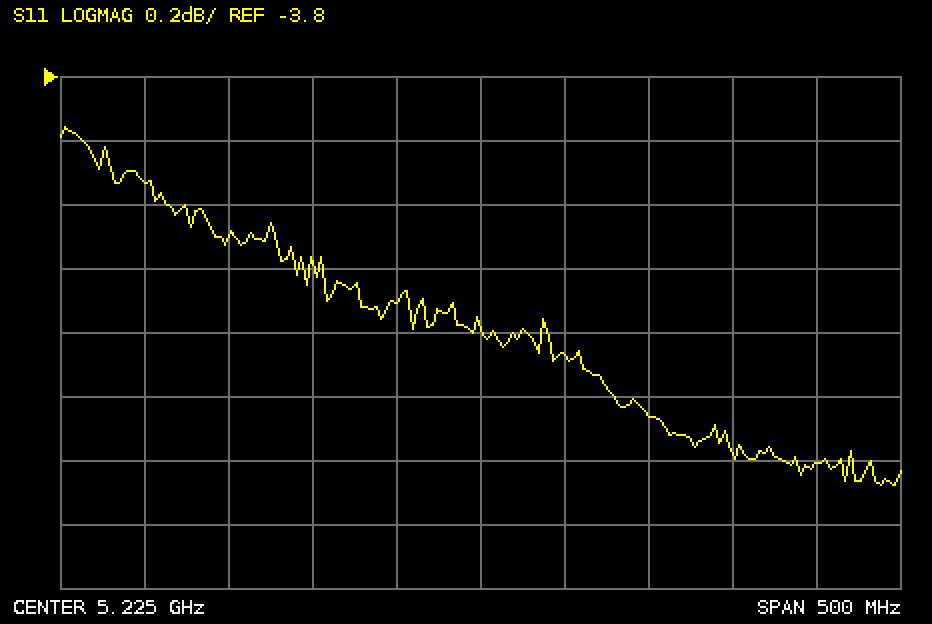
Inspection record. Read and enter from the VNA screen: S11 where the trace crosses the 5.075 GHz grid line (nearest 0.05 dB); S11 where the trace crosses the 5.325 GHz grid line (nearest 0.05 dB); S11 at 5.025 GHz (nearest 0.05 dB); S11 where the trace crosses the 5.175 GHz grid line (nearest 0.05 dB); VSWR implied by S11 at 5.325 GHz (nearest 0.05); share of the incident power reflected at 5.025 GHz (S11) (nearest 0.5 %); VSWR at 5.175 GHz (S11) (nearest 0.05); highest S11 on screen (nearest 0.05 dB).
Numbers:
-4.30 dB
-4.85 dB
-4.15 dB
-4.50 dB
3.65
38.5 %
3.95
-3.95 dB
